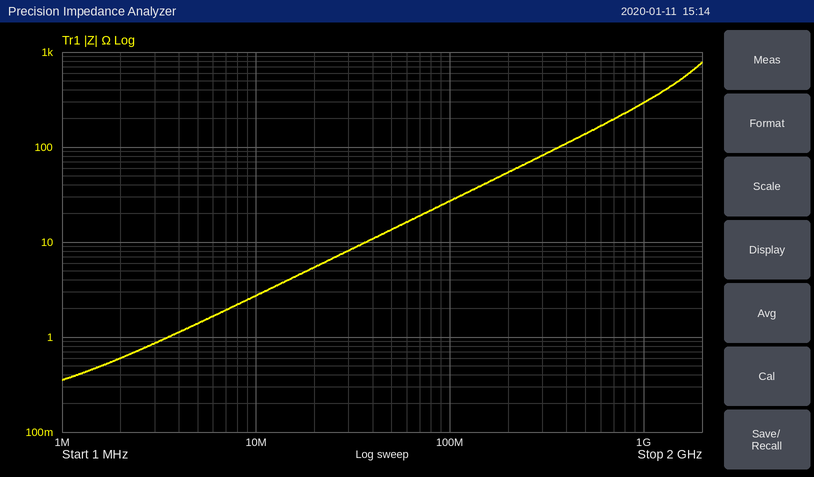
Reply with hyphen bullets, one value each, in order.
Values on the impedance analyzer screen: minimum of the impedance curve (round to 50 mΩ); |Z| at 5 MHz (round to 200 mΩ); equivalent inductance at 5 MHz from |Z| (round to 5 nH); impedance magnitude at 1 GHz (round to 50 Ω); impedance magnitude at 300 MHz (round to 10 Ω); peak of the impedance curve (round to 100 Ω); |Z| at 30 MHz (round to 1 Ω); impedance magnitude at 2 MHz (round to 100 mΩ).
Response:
- 350 mΩ
- 1.4 Ω
- 45 nH
- 300 Ω
- 80 Ω
- 800 Ω
- 8 Ω
- 600 mΩ
